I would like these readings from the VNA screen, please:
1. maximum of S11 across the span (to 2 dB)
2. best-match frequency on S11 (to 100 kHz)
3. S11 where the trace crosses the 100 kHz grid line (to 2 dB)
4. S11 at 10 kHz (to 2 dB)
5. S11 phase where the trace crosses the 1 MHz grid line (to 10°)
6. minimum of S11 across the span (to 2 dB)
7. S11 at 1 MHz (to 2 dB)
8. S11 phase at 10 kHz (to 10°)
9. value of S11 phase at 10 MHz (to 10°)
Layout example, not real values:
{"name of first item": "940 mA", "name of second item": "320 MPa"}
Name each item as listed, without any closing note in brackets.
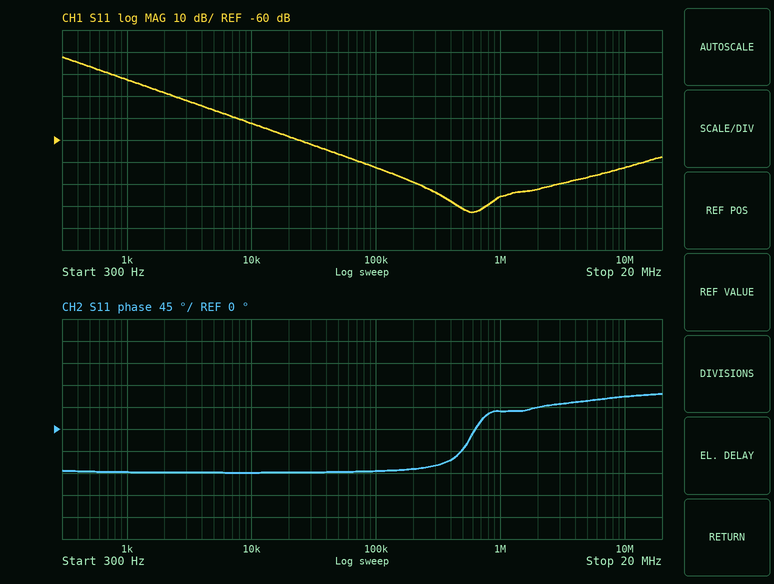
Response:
{"maximum of S11 across the span": "-22 dB", "best-match frequency on S11": "600 kHz", "S11 where the trace crosses the 100 kHz grid line": "-72 dB", "S11 at 10 kHz": "-52 dB", "S11 phase where the trace crosses the 1 MHz grid line": "40°", "minimum of S11 across the span": "-92 dB", "S11 at 1 MHz": "-86 dB", "S11 phase at 10 kHz": "-90°", "value of S11 phase at 10 MHz": "70°"}
